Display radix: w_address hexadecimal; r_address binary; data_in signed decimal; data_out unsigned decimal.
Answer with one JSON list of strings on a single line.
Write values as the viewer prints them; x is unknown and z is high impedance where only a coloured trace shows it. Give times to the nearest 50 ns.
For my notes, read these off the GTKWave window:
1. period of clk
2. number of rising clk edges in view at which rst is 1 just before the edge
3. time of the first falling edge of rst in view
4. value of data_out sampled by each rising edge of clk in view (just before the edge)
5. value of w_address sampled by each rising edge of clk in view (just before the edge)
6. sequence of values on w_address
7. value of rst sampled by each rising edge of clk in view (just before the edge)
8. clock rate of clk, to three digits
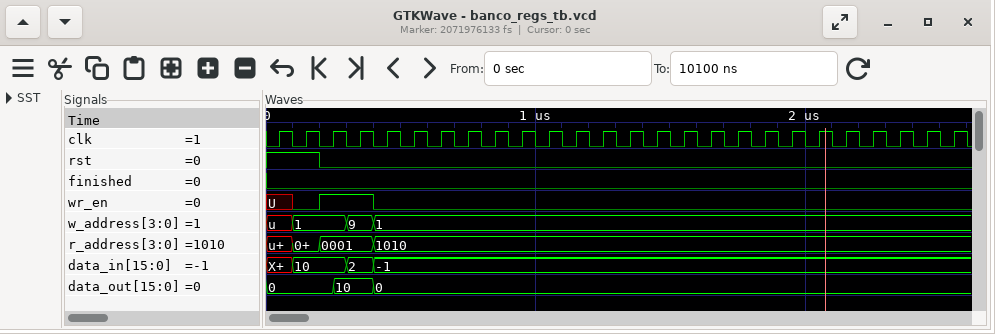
["100 ns", "2", "200 ns", "0, 0, 0, 10, 0, 0, 0, 0, 0, 0, 0, 0, 0, 0, 0, 0, 0, 0, 0, 0, 0, 0, 0, 0, 0, 0", "u, 1, 1, 9, 1, 1, 1, 1, 1, 1, 1, 1, 1, 1, 1, 1, 1, 1, 1, 1, 1, 1, 1, 1, 1, 1", "u, 1, 9, 1", "1 1 0 0 0 0 0 0 0 0 0 0 0 0 0 0 0 0 0 0 0 0 0 0 0 0", "10.0 MHz"]
